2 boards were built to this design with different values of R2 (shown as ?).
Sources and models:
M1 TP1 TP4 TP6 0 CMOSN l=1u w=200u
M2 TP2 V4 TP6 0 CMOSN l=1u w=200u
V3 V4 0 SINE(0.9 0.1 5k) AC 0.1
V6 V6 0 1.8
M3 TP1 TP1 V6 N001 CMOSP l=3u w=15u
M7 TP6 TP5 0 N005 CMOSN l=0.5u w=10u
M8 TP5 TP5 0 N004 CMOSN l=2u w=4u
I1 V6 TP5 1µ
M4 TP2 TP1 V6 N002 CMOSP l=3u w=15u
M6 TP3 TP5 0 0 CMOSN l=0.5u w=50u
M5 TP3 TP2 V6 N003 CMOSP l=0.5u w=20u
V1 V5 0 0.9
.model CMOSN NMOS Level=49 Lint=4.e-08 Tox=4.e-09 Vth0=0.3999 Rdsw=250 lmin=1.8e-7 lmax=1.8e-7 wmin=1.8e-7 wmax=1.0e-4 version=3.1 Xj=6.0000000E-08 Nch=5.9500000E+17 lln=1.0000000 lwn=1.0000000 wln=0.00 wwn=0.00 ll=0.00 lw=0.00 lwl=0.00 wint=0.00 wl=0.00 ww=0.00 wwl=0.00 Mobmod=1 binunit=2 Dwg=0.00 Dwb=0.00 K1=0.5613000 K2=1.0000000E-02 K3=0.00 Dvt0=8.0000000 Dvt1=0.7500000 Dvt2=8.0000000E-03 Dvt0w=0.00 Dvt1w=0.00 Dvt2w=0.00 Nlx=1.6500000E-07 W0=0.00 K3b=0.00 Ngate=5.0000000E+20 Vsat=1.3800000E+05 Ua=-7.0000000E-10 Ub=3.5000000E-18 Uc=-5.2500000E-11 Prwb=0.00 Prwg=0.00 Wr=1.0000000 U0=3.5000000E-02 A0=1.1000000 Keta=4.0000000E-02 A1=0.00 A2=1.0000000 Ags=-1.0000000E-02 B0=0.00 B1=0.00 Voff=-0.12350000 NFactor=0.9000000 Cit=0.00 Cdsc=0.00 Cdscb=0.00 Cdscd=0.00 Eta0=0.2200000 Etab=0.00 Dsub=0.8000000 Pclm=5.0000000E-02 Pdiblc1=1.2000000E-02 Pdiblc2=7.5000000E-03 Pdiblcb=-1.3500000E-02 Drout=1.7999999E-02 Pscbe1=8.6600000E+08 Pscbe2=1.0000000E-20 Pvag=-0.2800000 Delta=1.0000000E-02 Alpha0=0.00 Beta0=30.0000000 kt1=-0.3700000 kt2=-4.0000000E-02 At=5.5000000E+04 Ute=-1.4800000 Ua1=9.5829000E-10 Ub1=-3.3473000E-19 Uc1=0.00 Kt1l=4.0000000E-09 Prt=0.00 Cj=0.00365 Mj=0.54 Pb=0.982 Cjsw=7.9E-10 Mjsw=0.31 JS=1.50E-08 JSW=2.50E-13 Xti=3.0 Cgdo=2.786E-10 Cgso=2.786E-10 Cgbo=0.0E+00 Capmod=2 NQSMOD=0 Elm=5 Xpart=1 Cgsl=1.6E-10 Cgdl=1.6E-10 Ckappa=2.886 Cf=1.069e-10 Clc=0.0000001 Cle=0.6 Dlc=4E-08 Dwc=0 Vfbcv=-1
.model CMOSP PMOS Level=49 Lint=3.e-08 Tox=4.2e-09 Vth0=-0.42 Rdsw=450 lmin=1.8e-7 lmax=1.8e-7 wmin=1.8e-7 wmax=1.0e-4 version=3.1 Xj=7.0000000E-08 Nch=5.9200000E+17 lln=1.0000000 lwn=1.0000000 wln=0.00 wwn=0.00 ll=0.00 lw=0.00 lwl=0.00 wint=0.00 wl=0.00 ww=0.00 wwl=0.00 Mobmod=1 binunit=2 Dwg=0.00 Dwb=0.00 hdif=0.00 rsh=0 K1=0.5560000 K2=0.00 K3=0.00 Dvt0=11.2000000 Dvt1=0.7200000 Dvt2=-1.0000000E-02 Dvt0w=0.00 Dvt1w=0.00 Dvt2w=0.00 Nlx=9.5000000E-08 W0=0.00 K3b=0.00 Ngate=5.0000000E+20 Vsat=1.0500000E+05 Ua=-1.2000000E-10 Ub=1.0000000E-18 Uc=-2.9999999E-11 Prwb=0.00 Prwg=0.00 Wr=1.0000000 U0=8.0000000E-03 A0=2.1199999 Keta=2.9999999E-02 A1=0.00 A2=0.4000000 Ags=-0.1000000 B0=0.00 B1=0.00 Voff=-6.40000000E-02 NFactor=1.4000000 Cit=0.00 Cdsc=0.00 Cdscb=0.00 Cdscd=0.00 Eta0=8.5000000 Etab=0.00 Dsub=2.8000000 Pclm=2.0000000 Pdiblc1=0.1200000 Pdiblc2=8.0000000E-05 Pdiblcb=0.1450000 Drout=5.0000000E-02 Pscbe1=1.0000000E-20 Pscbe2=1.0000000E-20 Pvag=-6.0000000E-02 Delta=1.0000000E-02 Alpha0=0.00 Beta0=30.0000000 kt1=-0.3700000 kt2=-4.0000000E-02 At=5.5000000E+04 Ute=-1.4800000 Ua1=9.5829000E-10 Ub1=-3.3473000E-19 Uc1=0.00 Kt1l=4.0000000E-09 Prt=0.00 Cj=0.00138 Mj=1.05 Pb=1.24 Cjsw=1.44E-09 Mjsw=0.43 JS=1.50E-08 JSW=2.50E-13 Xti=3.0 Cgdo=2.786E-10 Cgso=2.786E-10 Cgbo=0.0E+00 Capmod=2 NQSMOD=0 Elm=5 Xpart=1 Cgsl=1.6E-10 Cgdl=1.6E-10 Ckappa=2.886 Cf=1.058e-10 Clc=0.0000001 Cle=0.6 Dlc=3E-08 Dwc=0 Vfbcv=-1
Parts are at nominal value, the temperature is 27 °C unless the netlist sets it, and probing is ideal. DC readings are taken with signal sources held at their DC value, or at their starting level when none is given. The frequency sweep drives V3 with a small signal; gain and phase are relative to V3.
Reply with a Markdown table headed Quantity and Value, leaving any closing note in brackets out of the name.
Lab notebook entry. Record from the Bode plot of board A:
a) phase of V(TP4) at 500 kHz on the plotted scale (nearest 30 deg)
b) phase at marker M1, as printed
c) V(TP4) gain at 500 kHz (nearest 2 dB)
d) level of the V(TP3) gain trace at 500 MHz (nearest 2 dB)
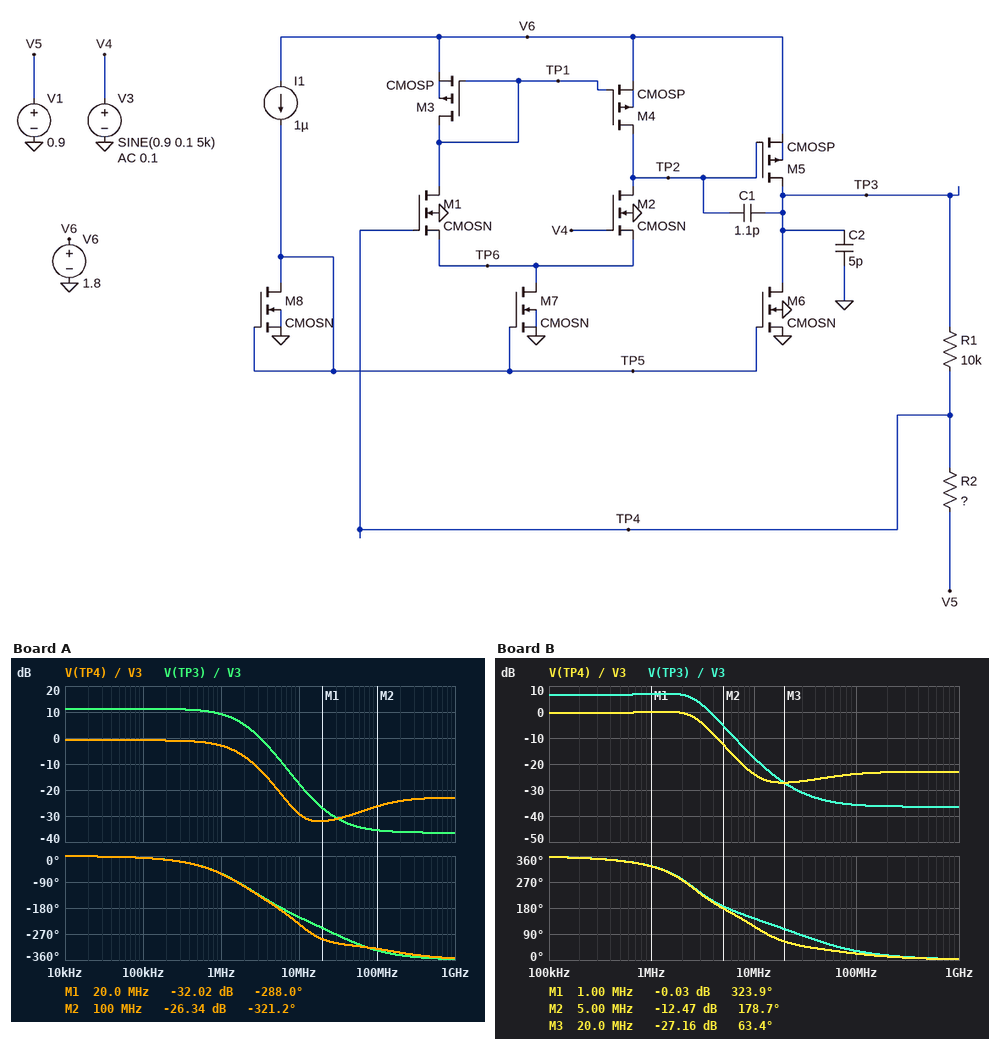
| Quantity | Value |
|---|---|
| phase of V(TP4) at 500 kHz on the plotted scale | -30 deg |
| phase at marker M1, as printed | -288.0 deg |
| V(TP4) gain at 500 kHz | -2 dB |
| level of the V(TP3) gain trace at 500 MHz | -36 dB |
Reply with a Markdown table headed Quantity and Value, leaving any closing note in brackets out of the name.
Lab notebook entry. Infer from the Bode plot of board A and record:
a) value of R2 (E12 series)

| Quantity | Value |
|---|---|
| value of R2 | 3.3 kΩ |
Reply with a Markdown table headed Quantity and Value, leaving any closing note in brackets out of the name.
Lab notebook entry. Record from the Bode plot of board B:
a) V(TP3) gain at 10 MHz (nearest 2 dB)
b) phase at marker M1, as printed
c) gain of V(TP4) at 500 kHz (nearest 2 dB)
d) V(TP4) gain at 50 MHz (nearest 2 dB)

| Quantity | Value |
|---|---|
| V(TP3) gain at 10 MHz | -18 dB |
| phase at marker M1, as printed | 323.9 deg |
| gain of V(TP4) at 500 kHz | 0 dB |
| V(TP4) gain at 50 MHz | -26 dB |
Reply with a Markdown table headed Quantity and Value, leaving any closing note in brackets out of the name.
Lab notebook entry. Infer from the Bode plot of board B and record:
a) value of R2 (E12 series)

| Quantity | Value |
|---|---|
| value of R2 | 8.2 kΩ |
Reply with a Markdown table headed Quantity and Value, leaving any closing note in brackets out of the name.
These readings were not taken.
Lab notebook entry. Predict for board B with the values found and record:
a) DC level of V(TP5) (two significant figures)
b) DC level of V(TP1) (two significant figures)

| Quantity | Value |
|---|---|
| DC level of V(TP5) | 380 mV |
| DC level of V(TP1) | 1.3 V |
